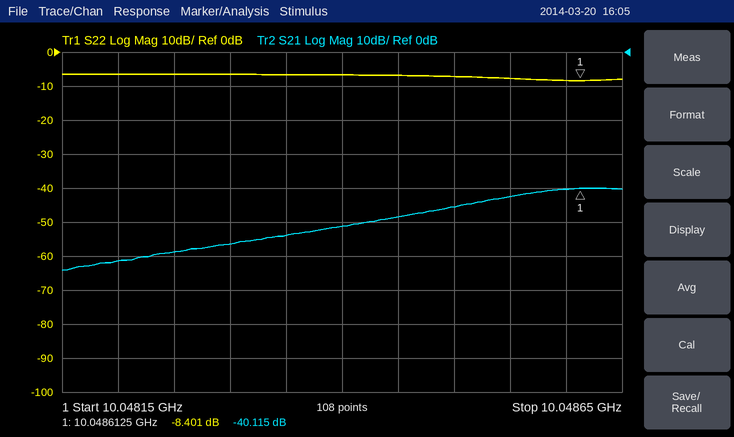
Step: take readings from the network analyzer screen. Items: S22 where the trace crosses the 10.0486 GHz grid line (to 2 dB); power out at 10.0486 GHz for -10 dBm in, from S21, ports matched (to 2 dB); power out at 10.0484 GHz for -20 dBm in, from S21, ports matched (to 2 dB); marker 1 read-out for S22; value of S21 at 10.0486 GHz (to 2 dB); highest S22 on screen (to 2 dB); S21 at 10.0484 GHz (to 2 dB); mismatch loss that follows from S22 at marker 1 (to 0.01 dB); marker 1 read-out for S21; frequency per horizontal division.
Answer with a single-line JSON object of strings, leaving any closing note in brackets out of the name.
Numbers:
{"S22 where the trace crosses the 10.0486 GHz grid line": "-8 dB", "power out at 10.0486 GHz for -10 dBm in, from S21, ports matched": "-50 dBm", "power out at 10.0484 GHz for -20 dBm in, from S21, ports matched": "-72 dBm", "marker 1 read-out for S22": "-8.401 dB", "value of S21 at 10.0486 GHz": "-40 dB", "highest S22 on screen": "-6 dB", "S21 at 10.0484 GHz": "-52 dB", "mismatch loss that follows from S22 at marker 1": "0.68 dB", "marker 1 read-out for S21": "-40.115 dB", "frequency per horizontal division": "50 kHz"}
